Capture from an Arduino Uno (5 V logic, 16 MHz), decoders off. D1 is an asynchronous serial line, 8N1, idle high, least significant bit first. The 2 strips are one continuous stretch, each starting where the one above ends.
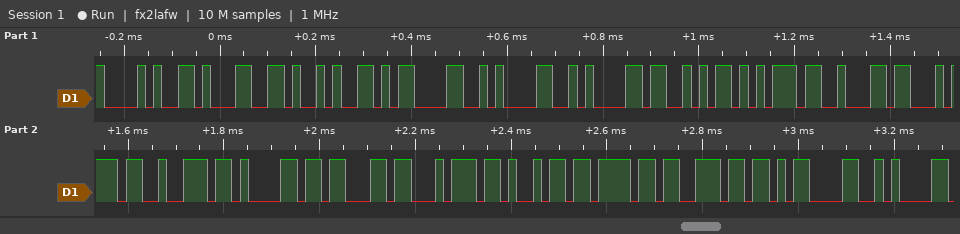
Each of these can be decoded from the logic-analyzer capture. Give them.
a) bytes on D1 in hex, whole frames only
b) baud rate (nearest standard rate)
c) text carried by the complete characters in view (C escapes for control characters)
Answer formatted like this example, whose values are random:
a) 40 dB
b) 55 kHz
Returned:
a) 28 31 29 0D 0A 0A 53 75 62 74 72 61 63 74 69 6F 6E 0D 0A
b) 57600 baud
c) "(1)\r\n\nSubtraction\r\n"
